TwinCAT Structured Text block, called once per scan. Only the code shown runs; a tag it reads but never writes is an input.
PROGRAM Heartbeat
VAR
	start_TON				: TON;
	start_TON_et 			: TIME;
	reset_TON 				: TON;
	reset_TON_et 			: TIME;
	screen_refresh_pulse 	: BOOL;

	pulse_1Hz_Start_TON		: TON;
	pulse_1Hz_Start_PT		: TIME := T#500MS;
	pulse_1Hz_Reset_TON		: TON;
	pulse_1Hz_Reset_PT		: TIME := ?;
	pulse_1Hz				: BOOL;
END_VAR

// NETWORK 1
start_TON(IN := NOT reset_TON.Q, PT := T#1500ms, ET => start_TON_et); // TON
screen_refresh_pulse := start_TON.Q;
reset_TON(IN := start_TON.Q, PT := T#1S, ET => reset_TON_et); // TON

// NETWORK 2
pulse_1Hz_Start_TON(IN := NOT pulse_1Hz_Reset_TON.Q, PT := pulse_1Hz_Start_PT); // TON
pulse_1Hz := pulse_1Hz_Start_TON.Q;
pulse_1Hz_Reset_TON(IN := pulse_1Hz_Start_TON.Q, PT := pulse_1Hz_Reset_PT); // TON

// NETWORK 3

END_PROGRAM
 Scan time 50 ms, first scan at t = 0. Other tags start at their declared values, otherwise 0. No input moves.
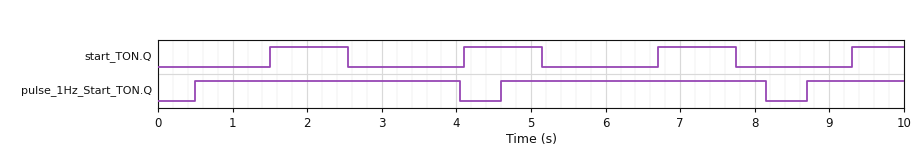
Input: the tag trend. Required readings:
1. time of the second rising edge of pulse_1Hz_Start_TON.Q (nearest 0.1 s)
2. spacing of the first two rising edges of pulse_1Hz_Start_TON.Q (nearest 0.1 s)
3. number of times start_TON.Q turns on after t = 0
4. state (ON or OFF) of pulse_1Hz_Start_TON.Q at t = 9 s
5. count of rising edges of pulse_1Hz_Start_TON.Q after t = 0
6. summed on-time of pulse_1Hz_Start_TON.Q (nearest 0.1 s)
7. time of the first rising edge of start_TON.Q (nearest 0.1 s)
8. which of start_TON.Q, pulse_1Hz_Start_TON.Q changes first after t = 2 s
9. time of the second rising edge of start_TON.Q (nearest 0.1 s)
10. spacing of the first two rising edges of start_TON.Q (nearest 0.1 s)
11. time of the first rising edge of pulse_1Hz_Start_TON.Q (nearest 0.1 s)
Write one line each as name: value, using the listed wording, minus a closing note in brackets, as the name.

time of the second rising edge of pulse_1Hz_Start_TON.Q: 4.6 s
spacing of the first two rising edges of pulse_1Hz_Start_TON.Q: 4.1 s
number of times start_TON.Q turns on after t = 0: 4
state (ON or OFF) of pulse_1Hz_Start_TON.Q at t = 9 s: ON
count of rising edges of pulse_1Hz_Start_TON.Q after t = 0: 3
summed on-time of pulse_1Hz_Start_TON.Q: 8.4 s
time of the first rising edge of start_TON.Q: 1.5 s
which of start_TON.Q, pulse_1Hz_Start_TON.Q changes first after t = 2 s: start_TON.Q
time of the second rising edge of start_TON.Q: 4.1 s
spacing of the first two rising edges of start_TON.Q: 2.6 s
time of the first rising edge of pulse_1Hz_Start_TON.Q: 0.5 s
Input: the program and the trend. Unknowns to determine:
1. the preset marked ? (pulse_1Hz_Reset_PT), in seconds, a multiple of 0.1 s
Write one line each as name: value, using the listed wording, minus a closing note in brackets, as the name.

the preset marked ? (pulse_1Hz_Reset_PT), in seconds, a multiple of 0.1 s: 3.5 s
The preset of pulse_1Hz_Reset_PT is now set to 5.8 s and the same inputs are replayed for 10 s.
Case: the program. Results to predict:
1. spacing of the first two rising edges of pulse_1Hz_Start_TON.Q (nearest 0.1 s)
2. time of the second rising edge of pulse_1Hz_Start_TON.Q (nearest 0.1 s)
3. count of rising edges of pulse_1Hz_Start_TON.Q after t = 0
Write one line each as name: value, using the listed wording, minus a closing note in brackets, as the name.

spacing of the first two rising edges of pulse_1Hz_Start_TON.Q: 6.4 s
time of the second rising edge of pulse_1Hz_Start_TON.Q: 6.9 s
count of rising edges of pulse_1Hz_Start_TON.Q after t = 0: 2
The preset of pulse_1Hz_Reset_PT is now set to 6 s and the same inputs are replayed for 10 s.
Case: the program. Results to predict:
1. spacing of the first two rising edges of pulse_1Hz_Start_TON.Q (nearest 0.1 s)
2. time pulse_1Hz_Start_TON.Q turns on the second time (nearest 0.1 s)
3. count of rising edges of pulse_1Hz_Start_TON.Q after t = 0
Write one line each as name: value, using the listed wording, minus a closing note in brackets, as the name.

spacing of the first two rising edges of pulse_1Hz_Start_TON.Q: 6.6 s
time pulse_1Hz_Start_TON.Q turns on the second time: 7.1 s
count of rising edges of pulse_1Hz_Start_TON.Q after t = 0: 2
